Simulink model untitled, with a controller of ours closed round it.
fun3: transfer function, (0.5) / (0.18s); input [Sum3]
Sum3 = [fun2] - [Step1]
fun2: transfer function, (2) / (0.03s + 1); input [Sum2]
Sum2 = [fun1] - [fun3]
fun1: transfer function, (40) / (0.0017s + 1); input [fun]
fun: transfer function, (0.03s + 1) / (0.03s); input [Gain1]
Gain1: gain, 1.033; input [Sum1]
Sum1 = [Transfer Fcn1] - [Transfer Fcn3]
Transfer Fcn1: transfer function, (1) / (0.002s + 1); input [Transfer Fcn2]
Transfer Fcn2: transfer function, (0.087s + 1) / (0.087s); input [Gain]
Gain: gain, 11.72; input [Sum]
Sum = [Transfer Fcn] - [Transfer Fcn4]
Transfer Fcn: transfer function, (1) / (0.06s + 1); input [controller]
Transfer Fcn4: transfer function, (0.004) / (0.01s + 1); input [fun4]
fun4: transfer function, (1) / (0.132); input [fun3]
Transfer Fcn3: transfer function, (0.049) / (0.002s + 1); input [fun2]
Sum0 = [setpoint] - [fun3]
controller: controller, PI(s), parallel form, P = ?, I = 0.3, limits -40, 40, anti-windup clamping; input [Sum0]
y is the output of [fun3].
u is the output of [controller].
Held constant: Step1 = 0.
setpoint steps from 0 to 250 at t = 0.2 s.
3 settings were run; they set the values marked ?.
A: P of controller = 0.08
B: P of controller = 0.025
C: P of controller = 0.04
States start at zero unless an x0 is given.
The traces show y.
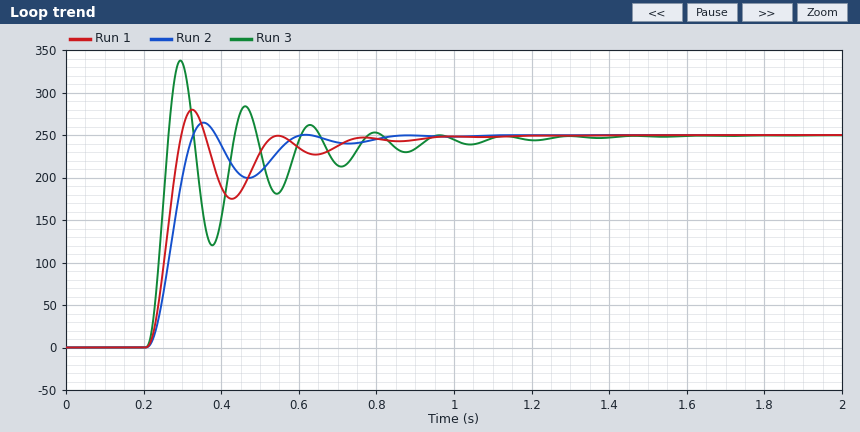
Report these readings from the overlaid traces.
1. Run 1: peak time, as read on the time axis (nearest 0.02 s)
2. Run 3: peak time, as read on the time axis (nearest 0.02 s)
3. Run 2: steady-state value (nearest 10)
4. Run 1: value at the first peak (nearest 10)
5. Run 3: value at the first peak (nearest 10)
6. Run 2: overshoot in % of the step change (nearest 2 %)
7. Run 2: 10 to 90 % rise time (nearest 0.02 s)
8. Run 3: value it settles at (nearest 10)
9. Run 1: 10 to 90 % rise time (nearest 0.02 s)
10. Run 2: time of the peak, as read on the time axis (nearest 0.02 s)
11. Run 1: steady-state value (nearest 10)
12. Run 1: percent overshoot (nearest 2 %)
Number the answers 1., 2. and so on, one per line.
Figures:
1. 0.32 s
2. 0.30 s
3. 250
4. 280
5. 340
6. 6 %
7. 0.08 s
8. 250
9. 0.06 s
10. 0.36 s
11. 250
12. 12 %
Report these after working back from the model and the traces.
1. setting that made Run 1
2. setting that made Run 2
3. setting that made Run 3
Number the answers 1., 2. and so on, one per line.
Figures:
1. C
2. B
3. A
